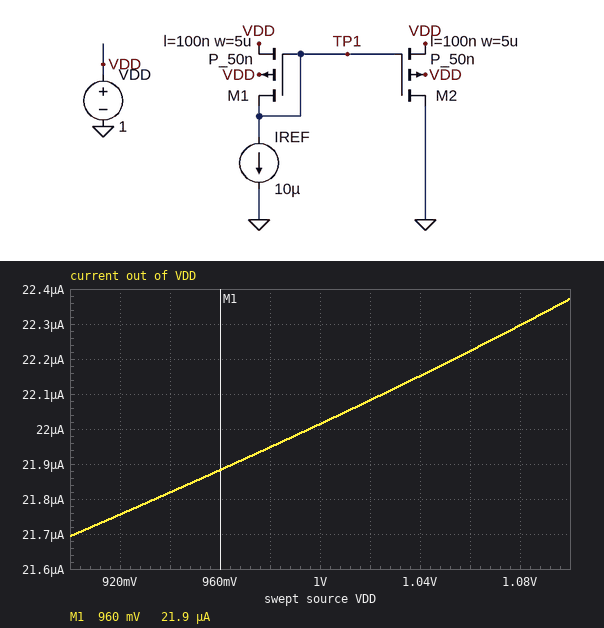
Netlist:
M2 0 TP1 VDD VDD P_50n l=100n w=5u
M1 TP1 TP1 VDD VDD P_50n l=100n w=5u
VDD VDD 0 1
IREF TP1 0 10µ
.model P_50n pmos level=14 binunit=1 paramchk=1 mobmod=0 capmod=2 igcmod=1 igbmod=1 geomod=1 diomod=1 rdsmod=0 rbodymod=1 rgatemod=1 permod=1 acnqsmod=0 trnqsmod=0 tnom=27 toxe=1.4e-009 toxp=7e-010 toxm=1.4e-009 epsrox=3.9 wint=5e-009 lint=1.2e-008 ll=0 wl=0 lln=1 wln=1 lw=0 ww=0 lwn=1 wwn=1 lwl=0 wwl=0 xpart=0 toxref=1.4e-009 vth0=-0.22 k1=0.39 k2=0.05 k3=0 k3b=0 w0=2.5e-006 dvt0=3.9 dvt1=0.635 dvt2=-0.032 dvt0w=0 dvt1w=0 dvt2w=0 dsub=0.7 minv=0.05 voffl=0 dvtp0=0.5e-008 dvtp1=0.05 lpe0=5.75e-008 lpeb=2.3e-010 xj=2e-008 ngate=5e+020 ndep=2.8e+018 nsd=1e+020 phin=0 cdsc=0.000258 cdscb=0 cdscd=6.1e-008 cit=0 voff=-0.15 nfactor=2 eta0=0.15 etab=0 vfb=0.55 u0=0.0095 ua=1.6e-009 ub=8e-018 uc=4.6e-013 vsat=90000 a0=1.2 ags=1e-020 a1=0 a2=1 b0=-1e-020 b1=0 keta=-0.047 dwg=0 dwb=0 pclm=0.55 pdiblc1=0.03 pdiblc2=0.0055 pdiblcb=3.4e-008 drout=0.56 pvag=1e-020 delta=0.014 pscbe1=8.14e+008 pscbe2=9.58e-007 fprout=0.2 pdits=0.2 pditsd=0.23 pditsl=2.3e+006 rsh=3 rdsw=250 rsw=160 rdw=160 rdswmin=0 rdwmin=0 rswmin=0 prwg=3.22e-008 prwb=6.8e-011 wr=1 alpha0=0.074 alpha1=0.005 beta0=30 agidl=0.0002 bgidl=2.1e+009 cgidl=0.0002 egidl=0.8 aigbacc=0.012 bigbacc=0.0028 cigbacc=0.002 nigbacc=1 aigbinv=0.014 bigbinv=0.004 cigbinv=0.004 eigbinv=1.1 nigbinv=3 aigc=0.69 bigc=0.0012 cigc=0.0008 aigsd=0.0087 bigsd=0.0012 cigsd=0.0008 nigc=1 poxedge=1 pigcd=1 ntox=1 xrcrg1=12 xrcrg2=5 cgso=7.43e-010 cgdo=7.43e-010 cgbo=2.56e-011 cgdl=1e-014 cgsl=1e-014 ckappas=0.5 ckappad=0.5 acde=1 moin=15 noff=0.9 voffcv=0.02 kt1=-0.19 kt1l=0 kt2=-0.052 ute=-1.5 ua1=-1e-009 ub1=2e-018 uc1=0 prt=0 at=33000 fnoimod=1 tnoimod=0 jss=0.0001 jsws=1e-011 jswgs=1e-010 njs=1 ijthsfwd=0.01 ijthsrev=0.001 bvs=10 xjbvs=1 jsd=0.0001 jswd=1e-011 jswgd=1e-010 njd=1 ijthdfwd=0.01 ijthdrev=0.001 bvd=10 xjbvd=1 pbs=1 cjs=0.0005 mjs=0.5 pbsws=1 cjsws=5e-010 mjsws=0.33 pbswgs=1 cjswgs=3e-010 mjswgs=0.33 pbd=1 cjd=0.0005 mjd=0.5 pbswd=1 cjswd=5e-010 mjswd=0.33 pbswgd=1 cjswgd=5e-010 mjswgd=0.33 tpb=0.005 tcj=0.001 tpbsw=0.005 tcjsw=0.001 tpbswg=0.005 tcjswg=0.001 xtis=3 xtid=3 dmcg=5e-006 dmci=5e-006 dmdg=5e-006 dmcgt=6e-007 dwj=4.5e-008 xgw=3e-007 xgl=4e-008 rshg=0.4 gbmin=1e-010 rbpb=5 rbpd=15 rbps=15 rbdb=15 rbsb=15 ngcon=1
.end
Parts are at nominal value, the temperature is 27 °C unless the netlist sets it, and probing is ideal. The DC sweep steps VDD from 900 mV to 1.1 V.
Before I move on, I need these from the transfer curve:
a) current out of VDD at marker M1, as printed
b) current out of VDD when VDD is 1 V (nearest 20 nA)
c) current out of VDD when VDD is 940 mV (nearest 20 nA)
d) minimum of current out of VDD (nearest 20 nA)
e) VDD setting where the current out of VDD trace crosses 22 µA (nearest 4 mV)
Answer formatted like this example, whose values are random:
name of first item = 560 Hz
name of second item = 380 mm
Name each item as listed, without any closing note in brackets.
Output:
current out of VDD at marker M1, as printed = 21.9 µA
current out of VDD when VDD is 1 V = 22.02 µA
current out of VDD when VDD is 940 mV = 21.82 µA
minimum of current out of VDD = 21.70 µA
VDD setting where the current out of VDD trace crosses 22 µA = 996 mV
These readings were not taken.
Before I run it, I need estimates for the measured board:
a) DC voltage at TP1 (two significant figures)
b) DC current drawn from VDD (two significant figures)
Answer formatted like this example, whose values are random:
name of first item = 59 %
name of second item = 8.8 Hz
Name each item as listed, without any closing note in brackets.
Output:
DC voltage at TP1 = 650 mV
DC current drawn from VDD = 22 µA
